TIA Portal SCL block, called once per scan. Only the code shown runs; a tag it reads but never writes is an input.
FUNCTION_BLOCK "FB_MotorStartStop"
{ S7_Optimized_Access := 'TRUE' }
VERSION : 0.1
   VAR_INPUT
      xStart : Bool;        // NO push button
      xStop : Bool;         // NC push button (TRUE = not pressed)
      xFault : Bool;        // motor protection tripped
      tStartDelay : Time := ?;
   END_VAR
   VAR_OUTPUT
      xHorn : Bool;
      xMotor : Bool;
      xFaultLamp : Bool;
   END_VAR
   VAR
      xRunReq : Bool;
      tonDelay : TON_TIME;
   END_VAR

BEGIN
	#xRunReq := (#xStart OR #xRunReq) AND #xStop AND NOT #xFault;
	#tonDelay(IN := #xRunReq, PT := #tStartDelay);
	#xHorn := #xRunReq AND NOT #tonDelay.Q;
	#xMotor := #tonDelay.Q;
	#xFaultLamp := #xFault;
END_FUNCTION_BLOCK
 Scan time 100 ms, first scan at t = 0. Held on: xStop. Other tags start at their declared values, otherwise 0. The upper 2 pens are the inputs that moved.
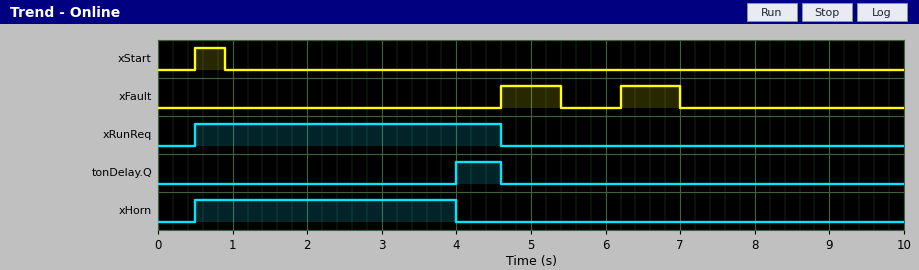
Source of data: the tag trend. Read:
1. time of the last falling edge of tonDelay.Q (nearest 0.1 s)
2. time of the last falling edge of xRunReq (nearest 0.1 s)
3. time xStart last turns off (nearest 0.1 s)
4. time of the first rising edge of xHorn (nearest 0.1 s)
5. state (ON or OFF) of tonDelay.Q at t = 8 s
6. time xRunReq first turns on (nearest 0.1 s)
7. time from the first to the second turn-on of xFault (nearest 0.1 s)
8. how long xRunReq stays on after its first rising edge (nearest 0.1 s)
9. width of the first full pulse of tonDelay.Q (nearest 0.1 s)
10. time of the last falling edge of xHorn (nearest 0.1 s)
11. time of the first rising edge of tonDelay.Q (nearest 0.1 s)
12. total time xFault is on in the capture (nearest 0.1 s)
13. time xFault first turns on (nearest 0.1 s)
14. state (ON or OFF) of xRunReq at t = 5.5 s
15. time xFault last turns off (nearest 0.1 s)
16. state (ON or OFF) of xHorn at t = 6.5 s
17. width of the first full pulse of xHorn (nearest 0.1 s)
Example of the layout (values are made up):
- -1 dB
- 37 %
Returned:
- 4.6 s
- 4.6 s
- 0.9 s
- 0.5 s
- OFF
- 0.5 s
- 1.6 s
- 4.1 s
- 0.6 s
- 4.0 s
- 4.0 s
- 1.6 s
- 4.6 s
- OFF
- 7.0 s
- OFF
- 3.5 s
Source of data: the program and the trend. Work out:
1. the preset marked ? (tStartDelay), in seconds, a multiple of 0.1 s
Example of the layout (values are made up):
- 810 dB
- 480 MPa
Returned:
- 3.5 s
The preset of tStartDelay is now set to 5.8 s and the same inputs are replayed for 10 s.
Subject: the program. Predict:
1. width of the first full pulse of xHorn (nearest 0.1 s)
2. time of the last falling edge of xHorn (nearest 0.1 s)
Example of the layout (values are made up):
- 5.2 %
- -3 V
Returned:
- 4.1 s
- 4.6 s
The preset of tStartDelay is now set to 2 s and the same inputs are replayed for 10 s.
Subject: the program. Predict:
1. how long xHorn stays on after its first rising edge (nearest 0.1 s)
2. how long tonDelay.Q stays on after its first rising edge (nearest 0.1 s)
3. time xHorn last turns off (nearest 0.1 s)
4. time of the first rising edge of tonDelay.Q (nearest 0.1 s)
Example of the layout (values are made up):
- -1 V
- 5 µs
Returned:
- 2.0 s
- 2.1 s
- 2.5 s
- 2.5 s
